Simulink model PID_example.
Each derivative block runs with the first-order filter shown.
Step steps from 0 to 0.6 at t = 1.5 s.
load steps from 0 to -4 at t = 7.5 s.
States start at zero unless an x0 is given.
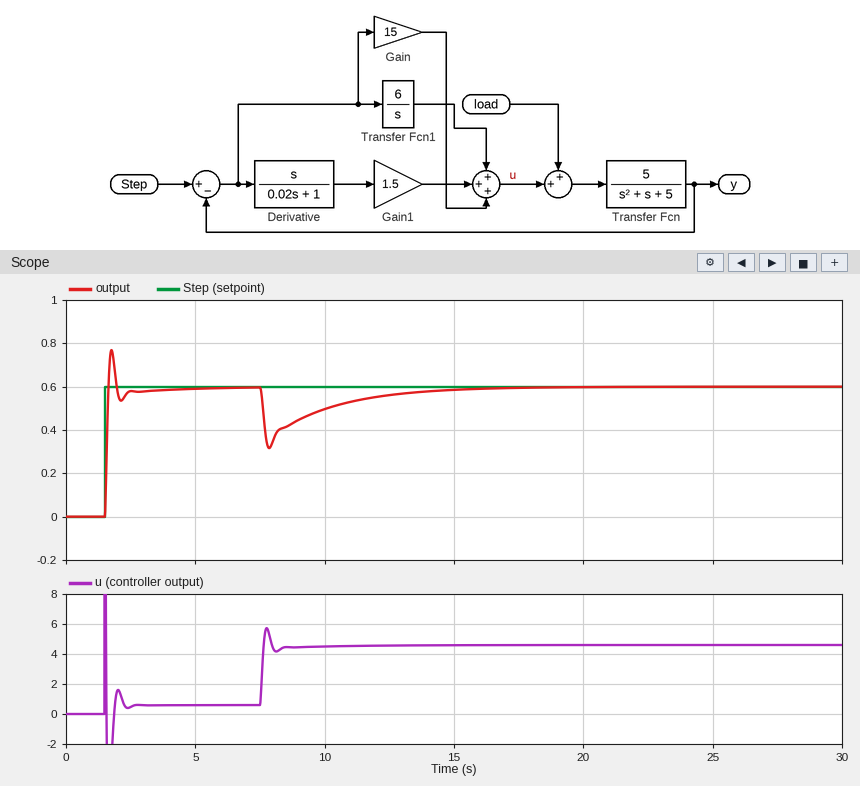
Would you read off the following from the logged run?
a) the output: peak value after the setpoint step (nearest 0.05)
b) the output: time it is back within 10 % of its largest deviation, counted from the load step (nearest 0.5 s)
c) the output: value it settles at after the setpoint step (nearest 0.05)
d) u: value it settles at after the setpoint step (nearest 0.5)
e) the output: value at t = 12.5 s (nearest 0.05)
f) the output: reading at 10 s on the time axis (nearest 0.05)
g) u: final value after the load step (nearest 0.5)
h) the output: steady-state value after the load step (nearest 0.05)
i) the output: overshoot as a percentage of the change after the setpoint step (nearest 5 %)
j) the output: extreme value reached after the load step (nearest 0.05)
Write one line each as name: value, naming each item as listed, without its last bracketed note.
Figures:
the output: peak value after the setpoint step: 0.75
the output: time it is back within 10 % of its largest deviation, counted from the load step: 6.0 s
the output: value it settles at after the setpoint step: 0.60
u: value it settles at after the setpoint step: 0.5
the output: value at t = 12.5 s: 0.55
the output: reading at 10 s on the time axis: 0.50
u: final value after the load step: 4.5
the output: steady-state value after the load step: 0.60
the output: overshoot as a percentage of the change after the setpoint step: 30 %
the output: extreme value reached after the load step: 0.30
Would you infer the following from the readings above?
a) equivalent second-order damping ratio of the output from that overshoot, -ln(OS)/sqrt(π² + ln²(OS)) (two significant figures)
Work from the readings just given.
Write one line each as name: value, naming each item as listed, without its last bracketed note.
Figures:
equivalent second-order damping ratio of the output from that overshoot, -ln(OS)/sqrt(π² + ln²(OS)): 0.36
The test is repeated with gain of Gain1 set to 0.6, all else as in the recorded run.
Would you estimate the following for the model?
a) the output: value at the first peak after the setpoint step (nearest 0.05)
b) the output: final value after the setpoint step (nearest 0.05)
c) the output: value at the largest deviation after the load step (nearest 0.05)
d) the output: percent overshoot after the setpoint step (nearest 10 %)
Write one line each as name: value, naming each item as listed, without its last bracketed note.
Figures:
the output: value at the first peak after the setpoint step: 0.90
the output: final value after the setpoint step: 0.60
the output: value at the largest deviation after the load step: 0.25
the output: percent overshoot after the setpoint step: 50 %
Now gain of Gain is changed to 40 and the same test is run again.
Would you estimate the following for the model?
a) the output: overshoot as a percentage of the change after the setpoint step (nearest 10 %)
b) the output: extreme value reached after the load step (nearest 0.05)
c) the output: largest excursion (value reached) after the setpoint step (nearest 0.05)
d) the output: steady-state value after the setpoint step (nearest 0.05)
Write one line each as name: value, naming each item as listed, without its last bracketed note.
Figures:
the output: overshoot as a percentage of the change after the setpoint step: 50 %
the output: extreme value reached after the load step: 0.45
the output: largest excursion (value reached) after the setpoint step: 0.90
the output: steady-state value after the setpoint step: 0.60
